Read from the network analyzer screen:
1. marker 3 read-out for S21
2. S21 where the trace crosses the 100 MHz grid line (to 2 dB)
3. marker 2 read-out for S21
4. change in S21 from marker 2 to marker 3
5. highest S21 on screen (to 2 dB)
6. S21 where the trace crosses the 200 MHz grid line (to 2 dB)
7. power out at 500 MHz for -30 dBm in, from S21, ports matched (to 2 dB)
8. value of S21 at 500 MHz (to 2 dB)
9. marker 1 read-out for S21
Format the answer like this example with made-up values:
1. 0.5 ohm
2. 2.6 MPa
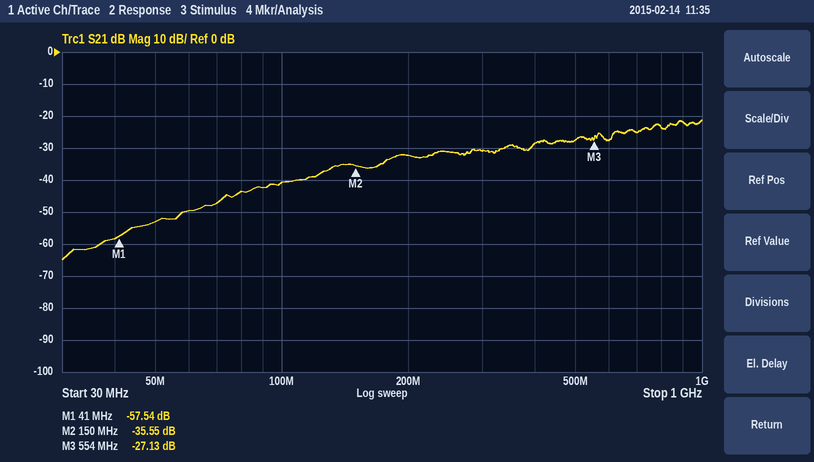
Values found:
1. -27.13 dB
2. -40 dB
3. -35.55 dB
4. 8.42 dB
5. -22 dB
6. -32 dB
7. -58 dBm
8. -28 dB
9. -57.54 dB
